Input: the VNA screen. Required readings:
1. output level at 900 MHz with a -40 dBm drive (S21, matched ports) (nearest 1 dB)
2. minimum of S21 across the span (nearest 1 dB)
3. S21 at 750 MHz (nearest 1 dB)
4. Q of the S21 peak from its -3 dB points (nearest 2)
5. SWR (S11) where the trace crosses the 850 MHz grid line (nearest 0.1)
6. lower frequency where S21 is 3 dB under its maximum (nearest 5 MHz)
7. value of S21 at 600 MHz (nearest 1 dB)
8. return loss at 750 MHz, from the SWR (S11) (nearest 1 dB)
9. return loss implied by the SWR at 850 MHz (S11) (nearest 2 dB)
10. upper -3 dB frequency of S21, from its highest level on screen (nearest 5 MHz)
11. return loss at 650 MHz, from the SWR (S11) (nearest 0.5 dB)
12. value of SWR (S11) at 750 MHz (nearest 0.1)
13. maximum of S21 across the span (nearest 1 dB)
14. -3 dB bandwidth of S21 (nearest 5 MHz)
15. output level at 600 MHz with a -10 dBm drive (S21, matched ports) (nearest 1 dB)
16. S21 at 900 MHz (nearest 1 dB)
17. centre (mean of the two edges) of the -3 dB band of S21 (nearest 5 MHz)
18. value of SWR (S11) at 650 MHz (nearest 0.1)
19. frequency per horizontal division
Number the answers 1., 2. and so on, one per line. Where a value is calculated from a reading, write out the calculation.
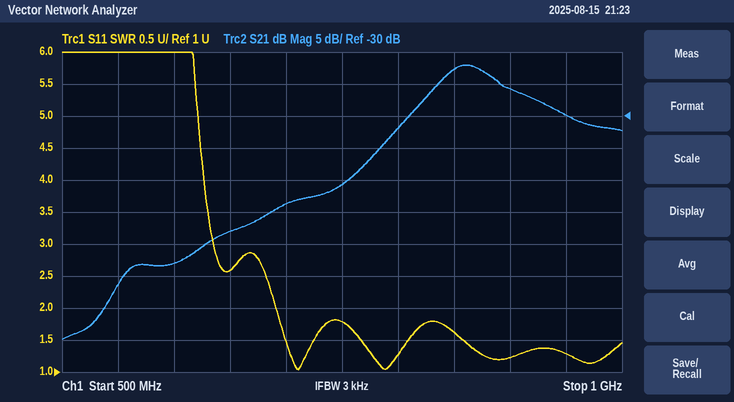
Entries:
1. -40 dBm + (-26 dB) = -66 dBm
2. -65 dB
3. -41 dB
4. 862.5 MHz / 55 MHz ≈ 16
5. 1.6
6. 835 MHz
7. -53 dB
8. −20 log10((1.8 − 1)/(1.8 + 1)) ≈ 11 dB
9. −20 log10((1.6 − 1)/(1.6 + 1)) ≈ 12.7 dB, so 12 dB to the nearest 2 dB
10. 890 MHz
11. −20 log10((2.6 − 1)/(2.6 + 1)) ≈ 7.0 dB
12. 1.8
13. -22 dB
14. 890 MHz − 835 MHz = 55 MHz
15. -10 dBm + (-53 dB) = -63 dBm
16. -26 dB
17. 865 MHz
18. 2.6
19. 50 MHz
